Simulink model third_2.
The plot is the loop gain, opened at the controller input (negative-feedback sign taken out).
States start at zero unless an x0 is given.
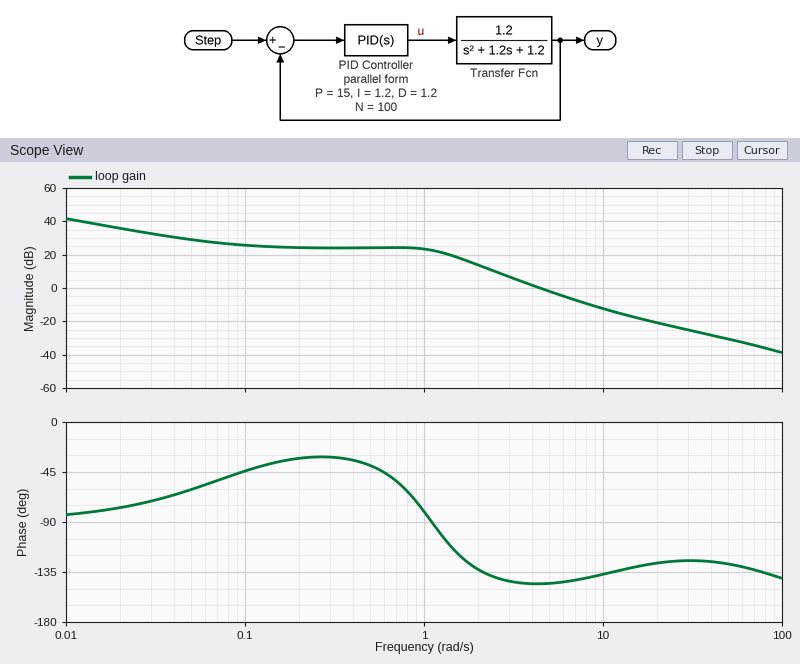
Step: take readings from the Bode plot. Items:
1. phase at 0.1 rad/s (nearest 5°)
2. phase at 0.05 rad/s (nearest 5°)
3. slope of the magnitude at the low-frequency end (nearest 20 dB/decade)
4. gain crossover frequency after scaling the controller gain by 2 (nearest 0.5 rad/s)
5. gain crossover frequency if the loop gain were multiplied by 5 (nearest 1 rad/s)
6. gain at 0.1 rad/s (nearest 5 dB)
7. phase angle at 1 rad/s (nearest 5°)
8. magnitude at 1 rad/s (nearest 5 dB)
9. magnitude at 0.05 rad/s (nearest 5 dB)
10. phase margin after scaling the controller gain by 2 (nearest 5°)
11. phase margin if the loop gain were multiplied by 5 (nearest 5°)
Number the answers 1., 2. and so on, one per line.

1. -45°
2. -60°
3. -20 dB/decade
4. 6.5 rad/s
5. 11 rad/s
6. 25 dB
7. -80°
8. 25 dB
9. 30 dB
10. 35°
11. 45°
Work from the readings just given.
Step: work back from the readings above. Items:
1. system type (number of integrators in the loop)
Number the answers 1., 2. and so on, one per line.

1. 1
